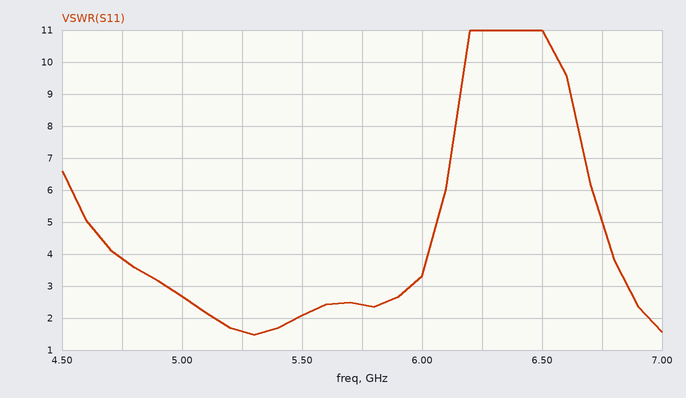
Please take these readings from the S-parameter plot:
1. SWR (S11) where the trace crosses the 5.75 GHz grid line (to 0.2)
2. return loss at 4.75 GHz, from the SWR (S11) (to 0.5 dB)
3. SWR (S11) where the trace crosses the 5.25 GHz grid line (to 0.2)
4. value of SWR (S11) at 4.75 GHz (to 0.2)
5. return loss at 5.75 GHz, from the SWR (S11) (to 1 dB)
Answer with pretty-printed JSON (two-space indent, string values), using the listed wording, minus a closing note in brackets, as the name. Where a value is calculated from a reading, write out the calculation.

{
  "SWR (S11) where the trace crosses the 5.75 GHz grid line": "2.4",
  "return loss at 4.75 GHz, from the SWR (S11)": "−20 log10((3.8 − 1)/(3.8 + 1)) ≈ 4.68 dB, so 4.5 dB to the nearest 0.5 dB",
  "SWR (S11) where the trace crosses the 5.25 GHz grid line": "1.6",
  "value of SWR (S11) at 4.75 GHz": "3.8",
  "return loss at 5.75 GHz, from the SWR (S11)": "−20 log10((2.4 − 1)/(2.4 + 1)) ≈ 8 dB"
}
